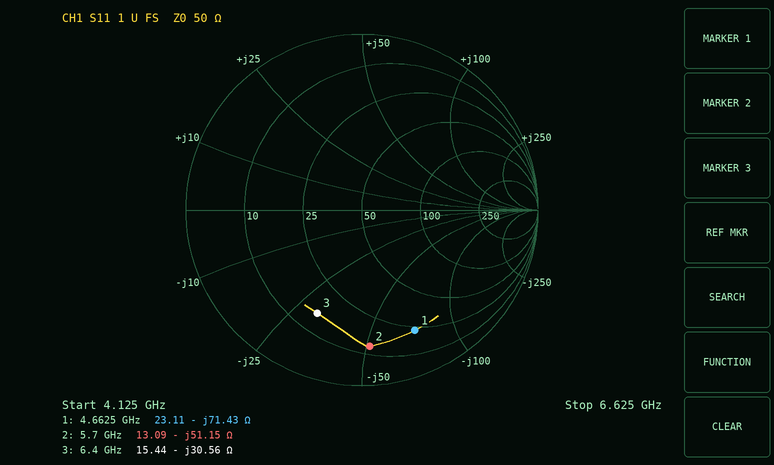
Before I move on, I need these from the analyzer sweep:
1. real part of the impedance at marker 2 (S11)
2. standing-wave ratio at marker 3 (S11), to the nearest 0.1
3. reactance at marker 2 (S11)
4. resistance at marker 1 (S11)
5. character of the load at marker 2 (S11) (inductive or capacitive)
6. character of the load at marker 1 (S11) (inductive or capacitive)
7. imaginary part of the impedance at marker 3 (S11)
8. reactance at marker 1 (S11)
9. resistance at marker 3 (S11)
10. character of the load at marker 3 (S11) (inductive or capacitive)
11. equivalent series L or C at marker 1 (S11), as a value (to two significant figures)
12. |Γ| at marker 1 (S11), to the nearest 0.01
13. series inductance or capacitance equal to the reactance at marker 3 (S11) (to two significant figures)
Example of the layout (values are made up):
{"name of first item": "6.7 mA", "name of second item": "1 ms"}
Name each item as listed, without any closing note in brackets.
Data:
{"real part of the impedance at marker 2": "13.09 Ω", "standing-wave ratio at marker 3 (S11), to the nearest 0.1": "4.5", "reactance at marker 2": "-51.15 Ω", "resistance at marker 1": "23.11 Ω", "character of the load at marker 2 (S11)": "capacitive", "character of the load at marker 1 (S11)": "capacitive", "imaginary part of the impedance at marker 3": "-30.56 Ω", "reactance at marker 1": "-71.43 Ω", "resistance at marker 3": "15.44 Ω", "character of the load at marker 3 (S11)": "capacitive", "equivalent series L or C at marker 1 (S11), as a value": "480 fF", "|Γ| at marker 1 (S11), to the nearest 0.01": "0.75", "series inductance or capacitance equal to the reactance at marker 3 (S11)": "810 fF"}
